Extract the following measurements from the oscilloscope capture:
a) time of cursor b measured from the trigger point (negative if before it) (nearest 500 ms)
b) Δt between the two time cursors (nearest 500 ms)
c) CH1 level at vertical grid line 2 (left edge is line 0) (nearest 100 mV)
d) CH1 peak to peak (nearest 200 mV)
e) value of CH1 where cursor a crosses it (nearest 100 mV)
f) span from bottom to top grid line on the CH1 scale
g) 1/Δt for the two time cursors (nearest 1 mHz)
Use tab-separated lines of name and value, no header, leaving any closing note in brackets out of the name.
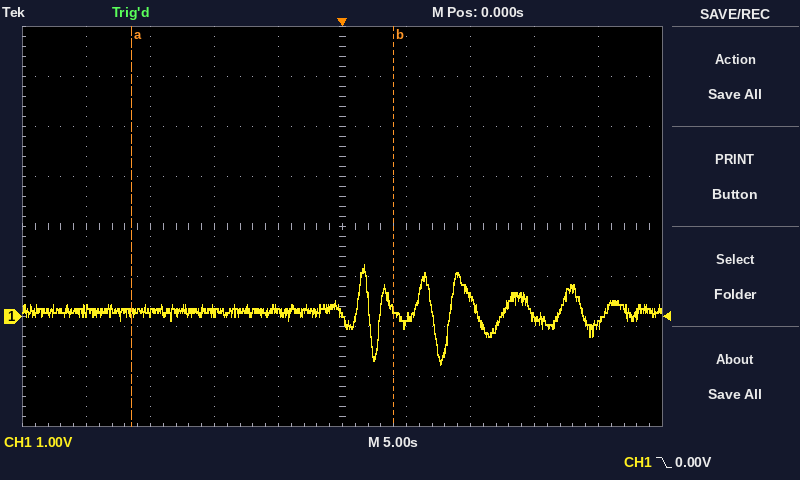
time of cursor b measured from the trigger point (negative if before it)	+4.0 s
Δt between the two time cursors	20.5 s
CH1 level at vertical grid line 2 (left edge is line 0)	100 mV
CH1 peak to peak	2.0 V
value of CH1 where cursor a crosses it	100 mV
span from bottom to top grid line on the CH1 scale	8 V
1/Δt for the two time cursors	49 mHz
